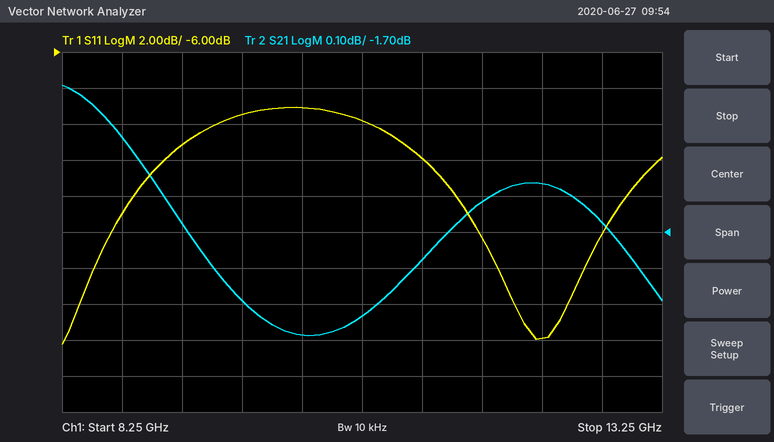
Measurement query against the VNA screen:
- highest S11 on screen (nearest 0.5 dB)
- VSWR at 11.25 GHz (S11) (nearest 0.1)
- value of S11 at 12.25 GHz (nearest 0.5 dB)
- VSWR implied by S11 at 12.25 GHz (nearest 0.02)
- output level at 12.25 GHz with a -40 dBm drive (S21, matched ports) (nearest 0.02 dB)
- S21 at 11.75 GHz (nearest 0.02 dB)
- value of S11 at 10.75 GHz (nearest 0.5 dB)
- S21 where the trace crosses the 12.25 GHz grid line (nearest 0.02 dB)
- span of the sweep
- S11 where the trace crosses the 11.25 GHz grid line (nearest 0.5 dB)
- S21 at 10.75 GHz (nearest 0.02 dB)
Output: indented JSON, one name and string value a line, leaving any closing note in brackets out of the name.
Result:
{
  "highest S11 on screen": "-9.0 dB",
  "VSWR at 11.25 GHz (S11)": "1.7",
  "value of S11 at 12.25 GHz": "-22.0 dB",
  "VSWR implied by S11 at 12.25 GHz": "1.18",
  "output level at 12.25 GHz with a -40 dBm drive (S21, matched ports)": "-41.56 dBm",
  "S21 at 11.75 GHz": "-1.62 dB",
  "value of S11 at 10.75 GHz": "-10.0 dB",
  "S21 where the trace crosses the 12.25 GHz grid line": "-1.56 dB",
  "span of the sweep": "5 GHz",
  "S11 where the trace crosses the 11.25 GHz grid line": "-12.0 dB",
  "S21 at 10.75 GHz": "-1.94 dB"
}
